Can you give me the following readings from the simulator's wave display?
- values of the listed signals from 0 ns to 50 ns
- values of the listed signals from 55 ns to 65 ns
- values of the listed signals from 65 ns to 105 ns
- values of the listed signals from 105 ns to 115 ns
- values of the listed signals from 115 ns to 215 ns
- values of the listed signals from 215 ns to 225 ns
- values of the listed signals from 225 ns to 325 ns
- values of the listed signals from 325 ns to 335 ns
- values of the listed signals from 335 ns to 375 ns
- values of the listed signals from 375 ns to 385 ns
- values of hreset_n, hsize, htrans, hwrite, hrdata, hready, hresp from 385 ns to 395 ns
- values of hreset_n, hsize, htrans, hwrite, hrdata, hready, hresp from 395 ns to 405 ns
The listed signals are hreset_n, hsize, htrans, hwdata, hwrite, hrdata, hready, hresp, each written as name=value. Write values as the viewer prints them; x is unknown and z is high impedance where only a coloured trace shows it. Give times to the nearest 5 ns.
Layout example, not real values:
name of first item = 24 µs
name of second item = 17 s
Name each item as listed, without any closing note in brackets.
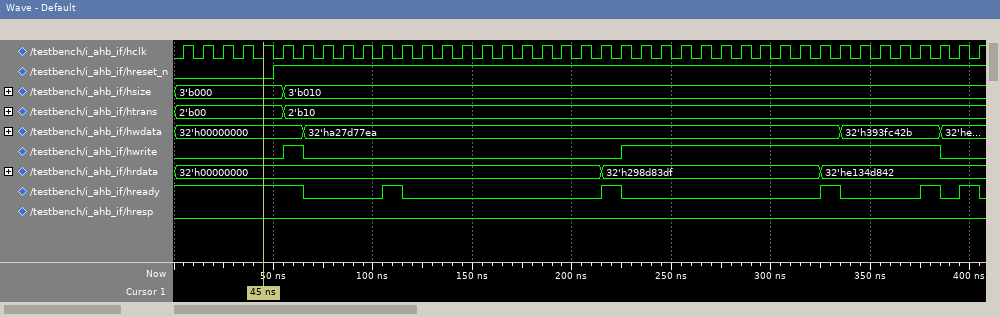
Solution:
values of the listed signals from 0 ns to 50 ns = hreset_n=0, hsize=3'b000, htrans=2'b00, hwdata=32'h00000000, hwrite=0, hrdata=32'h00000000, hready=1, hresp=0
values of the listed signals from 55 ns to 65 ns = hreset_n=1, hsize=3'b010, htrans=2'b10, hwdata=32'h00000000, hwrite=1, hrdata=32'h00000000, hready=1, hresp=0
values of the listed signals from 65 ns to 105 ns = hreset_n=1, hsize=3'b010, htrans=2'b10, hwdata=32'ha27d77ea, hwrite=0, hrdata=32'h00000000, hready=0, hresp=0
values of the listed signals from 105 ns to 115 ns = hreset_n=1, hsize=3'b010, htrans=2'b10, hwdata=32'ha27d77ea, hwrite=0, hrdata=32'h00000000, hready=1, hresp=0
values of the listed signals from 115 ns to 215 ns = hreset_n=1, hsize=3'b010, htrans=2'b10, hwdata=32'ha27d77ea, hwrite=0, hrdata=32'h00000000, hready=0, hresp=0
values of the listed signals from 215 ns to 225 ns = hreset_n=1, hsize=3'b010, htrans=2'b10, hwdata=32'ha27d77ea, hwrite=0, hrdata=32'h298d83df, hready=1, hresp=0
values of the listed signals from 225 ns to 325 ns = hreset_n=1, hsize=3'b010, htrans=2'b10, hwdata=32'ha27d77ea, hwrite=1, hrdata=32'h298d83df, hready=0, hresp=0
values of the listed signals from 325 ns to 335 ns = hreset_n=1, hsize=3'b010, htrans=2'b10, hwdata=32'ha27d77ea, hwrite=1, hrdata=32'he134d842, hready=1, hresp=0
values of the listed signals from 335 ns to 375 ns = hreset_n=1, hsize=3'b010, htrans=2'b10, hwdata=32'h393fc42b, hwrite=1, hrdata=32'he134d842, hready=0, hresp=0
values of the listed signals from 375 ns to 385 ns = hreset_n=1, hsize=3'b010, htrans=2'b10, hwdata=32'h393fc42b, hwrite=1, hrdata=32'he134d842, hready=1, hresp=0
values of hreset_n, hsize, htrans, hwrite, hrdata, hready, hresp from 385 ns to 395 ns = hreset_n=1, hsize=3'b010, htrans=2'b10, hwrite=0, hrdata=32'he134d842, hready=0, hresp=0
values of hreset_n, hsize, htrans, hwrite, hrdata, hready, hresp from 395 ns to 405 ns = hreset_n=1, hsize=3'b010, htrans=2'b10, hwrite=0, hrdata=32'he134d842, hready=1, hresp=0
